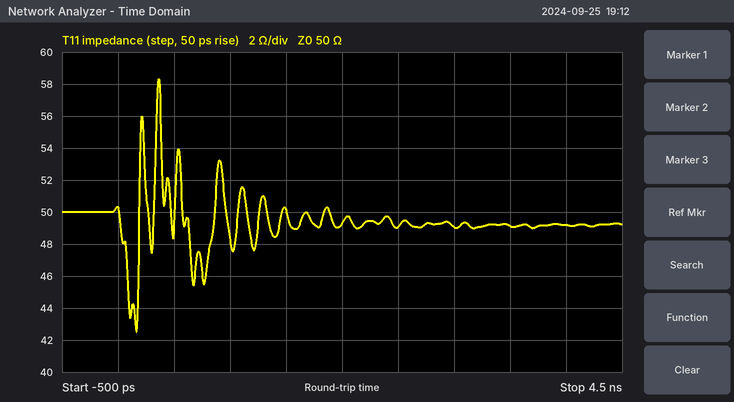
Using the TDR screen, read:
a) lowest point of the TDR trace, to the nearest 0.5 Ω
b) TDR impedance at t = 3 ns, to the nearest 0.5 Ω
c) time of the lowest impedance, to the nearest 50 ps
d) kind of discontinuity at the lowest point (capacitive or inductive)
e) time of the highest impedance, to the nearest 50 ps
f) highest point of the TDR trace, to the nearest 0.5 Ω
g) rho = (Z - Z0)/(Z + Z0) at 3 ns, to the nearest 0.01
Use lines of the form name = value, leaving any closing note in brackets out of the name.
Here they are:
lowest point of the TDR trace, to the nearest 0.5 Ω = 42.5 Ω
TDR impedance at t = 3 ns, to the nearest 0.5 Ω = 49.0 Ω
time of the lowest impedance, to the nearest 50 ps = 150 ps
kind of discontinuity at the lowest point = capacitive
time of the highest impedance, to the nearest 50 ps = 350 ps
highest point of the TDR trace, to the nearest 0.5 Ω = 58.5 Ω
rho = (Z - Z0)/(Z + Z0) at 3 ns, to the nearest 0.01 = -0.01
